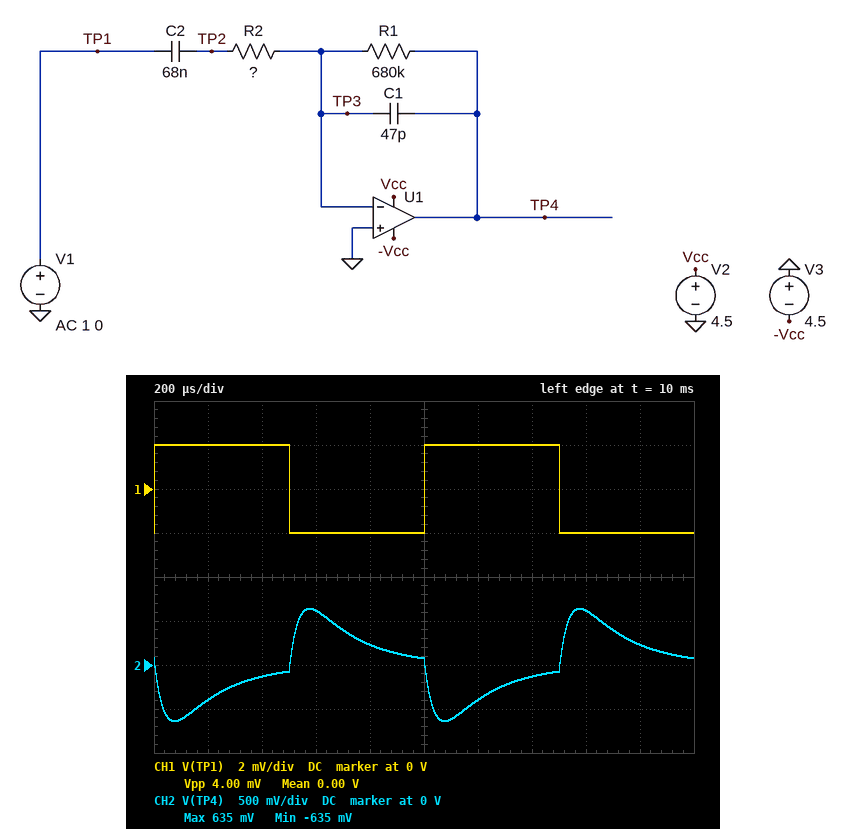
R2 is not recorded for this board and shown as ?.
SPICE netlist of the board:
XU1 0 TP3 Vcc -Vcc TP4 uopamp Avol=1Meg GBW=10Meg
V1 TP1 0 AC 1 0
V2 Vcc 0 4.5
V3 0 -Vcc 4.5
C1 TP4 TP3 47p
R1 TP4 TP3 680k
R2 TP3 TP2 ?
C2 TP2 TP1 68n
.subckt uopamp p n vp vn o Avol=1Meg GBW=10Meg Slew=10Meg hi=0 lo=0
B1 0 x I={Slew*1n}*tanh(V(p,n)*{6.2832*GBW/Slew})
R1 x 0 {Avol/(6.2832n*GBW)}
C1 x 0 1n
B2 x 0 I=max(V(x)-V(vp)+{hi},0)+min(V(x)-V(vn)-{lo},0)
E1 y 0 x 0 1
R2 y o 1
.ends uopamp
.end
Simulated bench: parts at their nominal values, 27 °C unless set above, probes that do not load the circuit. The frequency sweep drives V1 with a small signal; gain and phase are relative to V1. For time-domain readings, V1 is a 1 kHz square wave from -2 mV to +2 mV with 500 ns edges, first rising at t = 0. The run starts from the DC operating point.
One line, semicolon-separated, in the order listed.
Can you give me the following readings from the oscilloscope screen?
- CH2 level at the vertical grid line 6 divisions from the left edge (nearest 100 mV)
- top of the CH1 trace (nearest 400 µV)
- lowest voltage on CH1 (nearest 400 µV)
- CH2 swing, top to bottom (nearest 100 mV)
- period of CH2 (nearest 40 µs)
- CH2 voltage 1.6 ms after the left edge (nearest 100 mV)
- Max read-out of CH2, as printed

-400 mV; 2.0 mV; -2.0 mV; 1.3 V; 1.00 ms; 600 mV; 635 mV
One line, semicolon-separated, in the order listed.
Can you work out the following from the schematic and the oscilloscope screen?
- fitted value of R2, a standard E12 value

2.7 kΩ
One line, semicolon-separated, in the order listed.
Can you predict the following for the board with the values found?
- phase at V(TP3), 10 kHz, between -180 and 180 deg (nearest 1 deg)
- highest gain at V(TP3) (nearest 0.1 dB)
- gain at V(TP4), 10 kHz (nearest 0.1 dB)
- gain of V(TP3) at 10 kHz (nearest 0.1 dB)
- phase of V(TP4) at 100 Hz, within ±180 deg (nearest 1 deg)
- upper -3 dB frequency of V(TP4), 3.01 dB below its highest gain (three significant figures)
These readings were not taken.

28 deg; -19.1 dB; 40.2 dB; -19.8 dB; -98 deg; 5.85 kHz
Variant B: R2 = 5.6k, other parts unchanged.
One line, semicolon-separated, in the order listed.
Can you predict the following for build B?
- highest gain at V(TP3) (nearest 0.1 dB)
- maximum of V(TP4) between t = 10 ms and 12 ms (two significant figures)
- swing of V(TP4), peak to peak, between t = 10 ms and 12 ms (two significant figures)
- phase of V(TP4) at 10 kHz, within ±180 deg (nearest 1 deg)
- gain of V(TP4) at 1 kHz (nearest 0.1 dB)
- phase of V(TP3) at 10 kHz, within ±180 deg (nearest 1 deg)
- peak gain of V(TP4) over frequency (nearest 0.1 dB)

-24.9 dB; 300 mV; 590 mV; 117 deg; 40.8 dB; 27 deg; 41.0 dB
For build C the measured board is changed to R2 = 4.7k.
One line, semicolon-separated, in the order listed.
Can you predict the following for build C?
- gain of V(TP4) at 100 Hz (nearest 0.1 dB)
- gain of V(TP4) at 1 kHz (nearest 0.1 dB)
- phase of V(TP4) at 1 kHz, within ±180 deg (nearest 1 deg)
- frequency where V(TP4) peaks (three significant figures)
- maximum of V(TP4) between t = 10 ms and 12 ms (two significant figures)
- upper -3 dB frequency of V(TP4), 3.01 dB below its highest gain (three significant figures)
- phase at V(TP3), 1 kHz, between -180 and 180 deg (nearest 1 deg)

29.1 dB; 42.1 dB; -166 deg; 1.52 kHz; 360 mV; 5.53 kHz; 104 deg
